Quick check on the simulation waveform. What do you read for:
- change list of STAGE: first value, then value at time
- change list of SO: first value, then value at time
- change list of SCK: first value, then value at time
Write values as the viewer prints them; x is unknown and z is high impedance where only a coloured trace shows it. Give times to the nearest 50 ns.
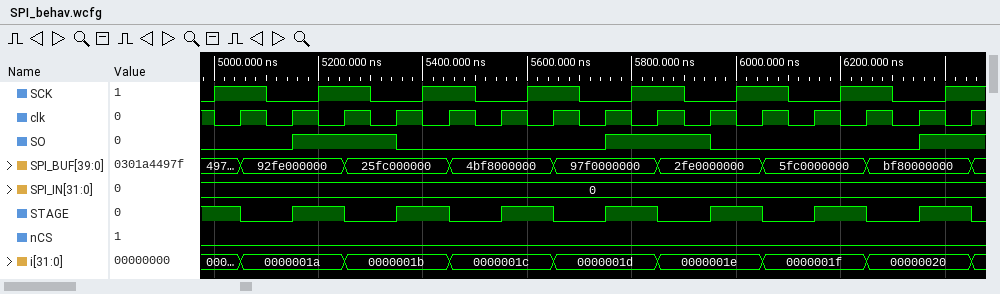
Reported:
1, 0 at 5050 ns, 1 at 5150 ns, 0 at 5250 ns, 1 at 5350 ns, 0 at 5450 ns, 1 at 5550 ns, 0 at 5650 ns, 1 at 5750 ns, 0 at 5850 ns, 1 at 5950 ns, 0 at 6050 ns, 1 at 6150 ns, 0 at 6250 ns, 1 at 6350 ns, 0 at 6450 ns
0, 1 at 5150 ns, 0 at 5350 ns, 1 at 5750 ns, 0 at 5950 ns, 1 at 6350 ns
0, 1 at 5000 ns, 0 at 5100 ns, 1 at 5200 ns, 0 at 5300 ns, 1 at 5400 ns, 0 at 5500 ns, 1 at 5600 ns, 0 at 5700 ns, 1 at 5800 ns, 0 at 5900 ns, 1 at 6000 ns, 0 at 6100 ns, 1 at 6200 ns, 0 at 6300 ns, 1 at 6400 ns
